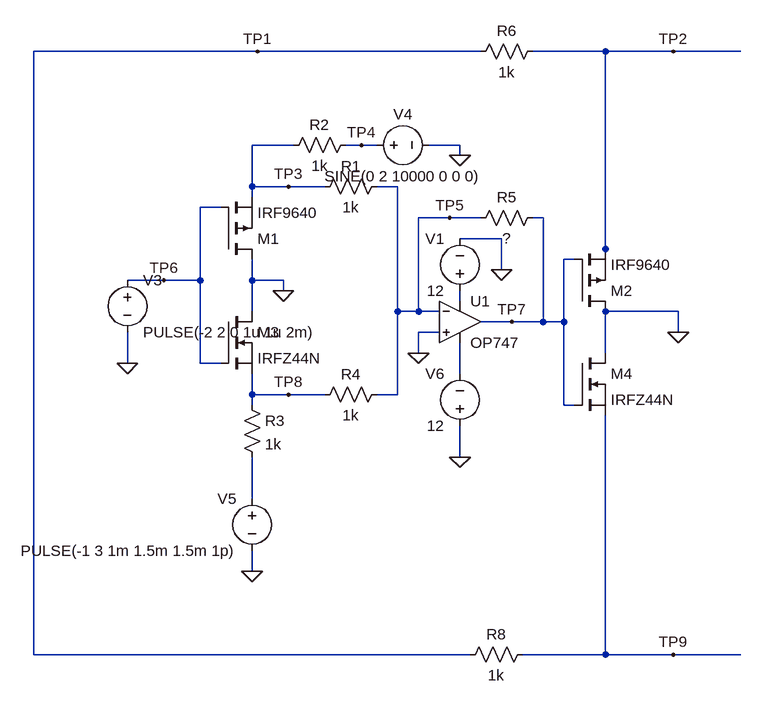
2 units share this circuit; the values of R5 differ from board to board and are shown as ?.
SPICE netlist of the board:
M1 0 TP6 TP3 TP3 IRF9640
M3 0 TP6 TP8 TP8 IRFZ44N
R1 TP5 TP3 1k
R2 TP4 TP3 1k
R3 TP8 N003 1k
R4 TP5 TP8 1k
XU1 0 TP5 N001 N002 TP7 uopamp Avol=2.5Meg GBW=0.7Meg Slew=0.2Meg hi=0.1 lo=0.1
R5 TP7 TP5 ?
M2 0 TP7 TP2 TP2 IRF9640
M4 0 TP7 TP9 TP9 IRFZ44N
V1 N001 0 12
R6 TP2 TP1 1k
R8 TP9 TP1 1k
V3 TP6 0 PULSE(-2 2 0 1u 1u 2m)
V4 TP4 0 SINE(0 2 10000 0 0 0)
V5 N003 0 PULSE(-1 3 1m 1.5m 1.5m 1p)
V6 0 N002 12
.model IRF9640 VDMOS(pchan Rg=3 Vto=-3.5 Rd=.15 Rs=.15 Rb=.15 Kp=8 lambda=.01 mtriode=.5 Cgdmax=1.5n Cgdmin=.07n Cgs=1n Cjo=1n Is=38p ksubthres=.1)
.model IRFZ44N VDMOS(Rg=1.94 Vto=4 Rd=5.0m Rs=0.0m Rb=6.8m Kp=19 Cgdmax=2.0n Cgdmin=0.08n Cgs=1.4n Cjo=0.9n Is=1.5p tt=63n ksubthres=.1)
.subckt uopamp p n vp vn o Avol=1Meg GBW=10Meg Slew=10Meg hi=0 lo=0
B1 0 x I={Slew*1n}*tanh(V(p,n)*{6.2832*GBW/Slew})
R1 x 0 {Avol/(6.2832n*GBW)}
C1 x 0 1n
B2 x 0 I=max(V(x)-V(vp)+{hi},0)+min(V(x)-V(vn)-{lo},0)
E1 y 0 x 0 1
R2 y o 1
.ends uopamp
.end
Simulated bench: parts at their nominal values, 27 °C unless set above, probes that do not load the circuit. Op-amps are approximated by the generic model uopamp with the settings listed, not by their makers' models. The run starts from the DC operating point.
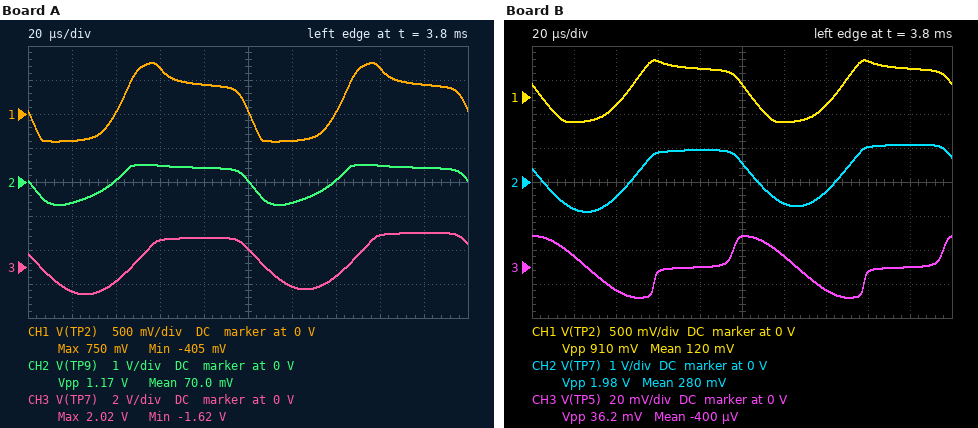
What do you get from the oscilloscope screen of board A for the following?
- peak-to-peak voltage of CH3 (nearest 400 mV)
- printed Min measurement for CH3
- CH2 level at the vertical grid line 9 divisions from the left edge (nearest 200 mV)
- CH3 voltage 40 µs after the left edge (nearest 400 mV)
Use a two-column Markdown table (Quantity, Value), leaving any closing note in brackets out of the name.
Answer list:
| Quantity | Value |
|---|---|
| peak-to-peak voltage of CH3 | 3.6 V |
| printed Min measurement for CH3 | -1.62 V |
| CH2 level at the vertical grid line 9 divisions from the left edge | 400 mV |
| CH3 voltage 40 µs after the left edge | -800 mV |
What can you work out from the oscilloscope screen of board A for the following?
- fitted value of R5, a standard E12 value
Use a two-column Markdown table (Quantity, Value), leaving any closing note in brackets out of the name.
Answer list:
| Quantity | Value |
|---|---|
| fitted value of R5, a standard E12 value | 2.2 kΩ |
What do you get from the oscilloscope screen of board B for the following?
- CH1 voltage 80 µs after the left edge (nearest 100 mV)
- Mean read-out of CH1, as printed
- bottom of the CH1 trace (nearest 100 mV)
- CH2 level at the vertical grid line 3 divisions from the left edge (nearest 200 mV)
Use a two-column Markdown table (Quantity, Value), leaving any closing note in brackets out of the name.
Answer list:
| Quantity | Value |
|---|---|
| CH1 voltage 80 µs after the left edge | 400 mV |
| Mean read-out of CH1, as printed | 120 mV |
| bottom of the CH1 trace | -400 mV |
| CH2 level at the vertical grid line 3 divisions from the left edge | 800 mV |
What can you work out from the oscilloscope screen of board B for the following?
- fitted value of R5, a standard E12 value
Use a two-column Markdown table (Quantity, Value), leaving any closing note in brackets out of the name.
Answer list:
| Quantity | Value |
|---|---|
| fitted value of R5, a standard E12 value | 1.2 kΩ |
